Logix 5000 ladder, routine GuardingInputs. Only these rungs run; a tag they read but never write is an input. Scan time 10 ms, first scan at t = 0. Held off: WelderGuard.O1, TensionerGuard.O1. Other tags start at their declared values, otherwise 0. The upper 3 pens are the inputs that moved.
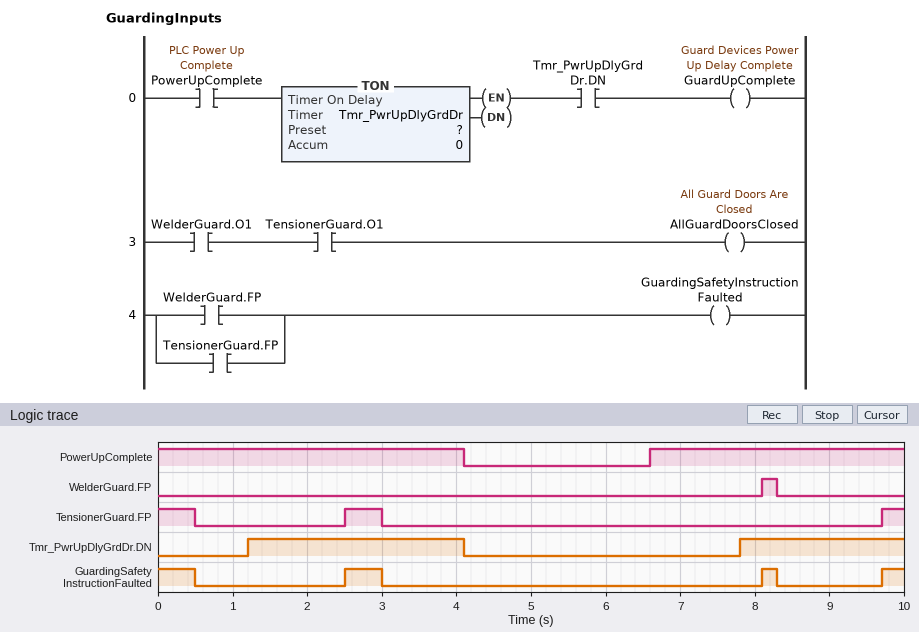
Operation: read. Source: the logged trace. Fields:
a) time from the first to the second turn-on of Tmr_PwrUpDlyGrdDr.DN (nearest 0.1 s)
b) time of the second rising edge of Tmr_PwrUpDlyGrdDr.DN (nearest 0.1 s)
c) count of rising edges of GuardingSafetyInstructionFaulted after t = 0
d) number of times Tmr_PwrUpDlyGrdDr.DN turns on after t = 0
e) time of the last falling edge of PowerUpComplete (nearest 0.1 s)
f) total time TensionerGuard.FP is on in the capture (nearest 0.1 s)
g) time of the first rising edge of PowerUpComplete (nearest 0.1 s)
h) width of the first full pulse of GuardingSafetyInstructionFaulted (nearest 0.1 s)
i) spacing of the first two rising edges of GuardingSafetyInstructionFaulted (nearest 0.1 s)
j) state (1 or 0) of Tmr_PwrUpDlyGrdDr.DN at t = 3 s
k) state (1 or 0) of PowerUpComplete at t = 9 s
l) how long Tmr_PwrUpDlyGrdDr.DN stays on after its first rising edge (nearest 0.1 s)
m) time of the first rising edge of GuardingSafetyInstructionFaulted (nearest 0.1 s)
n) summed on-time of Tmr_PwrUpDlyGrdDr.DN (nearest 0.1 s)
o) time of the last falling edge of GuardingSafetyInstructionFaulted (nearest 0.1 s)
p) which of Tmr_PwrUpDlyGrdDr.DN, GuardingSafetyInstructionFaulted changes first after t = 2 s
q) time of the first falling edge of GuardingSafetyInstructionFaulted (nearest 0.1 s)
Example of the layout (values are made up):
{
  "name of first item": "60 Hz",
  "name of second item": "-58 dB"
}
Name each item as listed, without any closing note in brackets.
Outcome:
{
  "time from the first to the second turn-on of Tmr_PwrUpDlyGrdDr.DN": "6.6 s",
  "time of the second rising edge of Tmr_PwrUpDlyGrdDr.DN": "7.8 s",
  "count of rising edges of GuardingSafetyInstructionFaulted after t = 0": "3",
  "number of times Tmr_PwrUpDlyGrdDr.DN turns on after t = 0": "2",
  "time of the last falling edge of PowerUpComplete": "4.1 s",
  "total time TensionerGuard.FP is on in the capture": "1.3 s",
  "time of the first rising edge of PowerUpComplete": "6.6 s",
  "width of the first full pulse of GuardingSafetyInstructionFaulted": "0.5 s",
  "spacing of the first two rising edges of GuardingSafetyInstructionFaulted": "5.6 s",
  "state (1 or 0) of Tmr_PwrUpDlyGrdDr.DN at t = 3 s": "1",
  "state (1 or 0) of PowerUpComplete at t = 9 s": "1",
  "how long Tmr_PwrUpDlyGrdDr.DN stays on after its first rising edge": "2.9 s",
  "time of the first rising edge of GuardingSafetyInstructionFaulted": "2.5 s",
  "summed on-time of Tmr_PwrUpDlyGrdDr.DN": "5.1 s",
  "time of the last falling edge of GuardingSafetyInstructionFaulted": "8.3 s",
  "which of Tmr_PwrUpDlyGrdDr.DN, GuardingSafetyInstructionFaulted changes first after t = 2 s": "GuardingSafetyInstructionFaulted",
  "time of the first falling edge of GuardingSafetyInstructionFaulted": "0.5 s"
}
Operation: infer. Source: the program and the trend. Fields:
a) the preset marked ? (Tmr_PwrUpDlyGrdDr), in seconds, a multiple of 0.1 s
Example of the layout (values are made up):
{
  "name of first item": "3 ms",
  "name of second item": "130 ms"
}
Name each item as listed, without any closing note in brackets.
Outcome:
{
  "the preset marked ? (Tmr_PwrUpDlyGrdDr), in seconds, a multiple of 0.1 s": "1.2 s"
}
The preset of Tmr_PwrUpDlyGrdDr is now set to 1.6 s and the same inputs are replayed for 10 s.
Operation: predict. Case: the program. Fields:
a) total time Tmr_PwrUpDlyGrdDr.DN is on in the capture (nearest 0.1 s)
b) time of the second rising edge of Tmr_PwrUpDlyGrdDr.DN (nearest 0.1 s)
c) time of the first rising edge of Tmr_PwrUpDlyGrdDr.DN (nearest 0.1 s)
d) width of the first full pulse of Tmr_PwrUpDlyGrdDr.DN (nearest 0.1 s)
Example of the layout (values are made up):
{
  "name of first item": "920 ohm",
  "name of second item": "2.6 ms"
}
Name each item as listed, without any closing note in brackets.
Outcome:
{
  "total time Tmr_PwrUpDlyGrdDr.DN is on in the capture": "4.3 s",
  "time of the second rising edge of Tmr_PwrUpDlyGrdDr.DN": "8.2 s",
  "time of the first rising edge of Tmr_PwrUpDlyGrdDr.DN": "1.6 s",
  "width of the first full pulse of Tmr_PwrUpDlyGrdDr.DN": "2.5 s"
}
